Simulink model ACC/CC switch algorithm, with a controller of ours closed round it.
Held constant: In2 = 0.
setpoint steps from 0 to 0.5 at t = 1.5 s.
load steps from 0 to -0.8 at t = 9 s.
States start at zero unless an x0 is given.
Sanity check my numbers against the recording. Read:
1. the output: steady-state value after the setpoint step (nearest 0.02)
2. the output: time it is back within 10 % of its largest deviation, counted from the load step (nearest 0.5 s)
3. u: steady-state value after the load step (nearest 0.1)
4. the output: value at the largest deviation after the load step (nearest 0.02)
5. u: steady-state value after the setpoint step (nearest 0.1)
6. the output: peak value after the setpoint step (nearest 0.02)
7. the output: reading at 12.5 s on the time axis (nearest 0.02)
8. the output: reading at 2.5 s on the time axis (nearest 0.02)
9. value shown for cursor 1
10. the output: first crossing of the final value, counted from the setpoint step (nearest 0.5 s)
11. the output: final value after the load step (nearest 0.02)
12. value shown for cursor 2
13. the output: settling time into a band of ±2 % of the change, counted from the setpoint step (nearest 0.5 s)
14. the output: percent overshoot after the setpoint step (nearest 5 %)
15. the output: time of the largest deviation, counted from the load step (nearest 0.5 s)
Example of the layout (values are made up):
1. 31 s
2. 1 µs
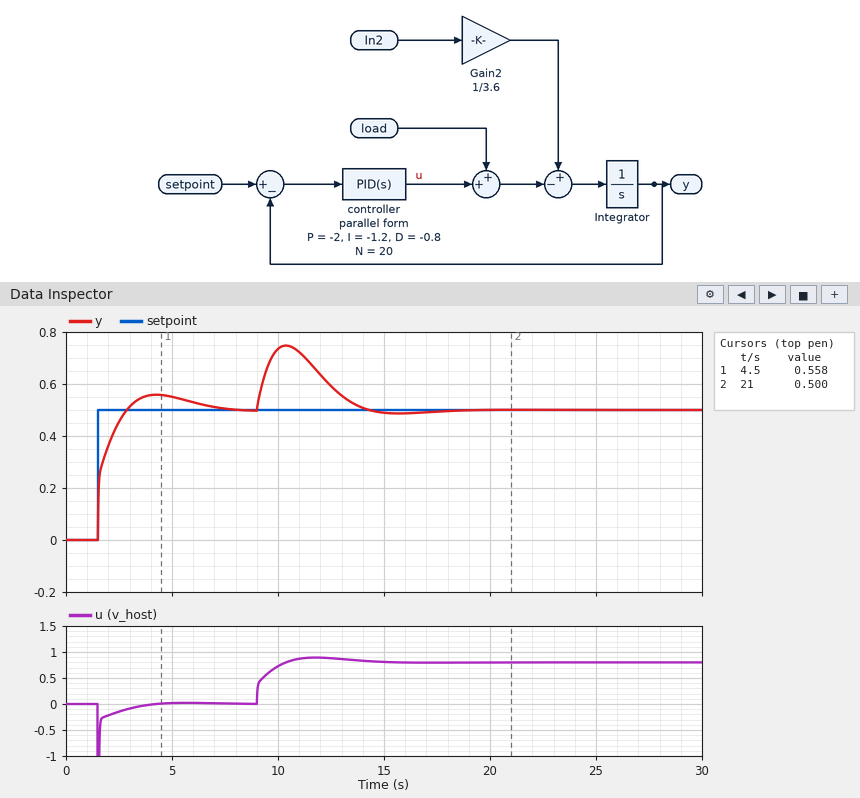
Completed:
1. 0.50
2. 4.5 s
3. 0.8
4. 0.74
5. 0.0
6. 0.56
7. 0.60
8. 0.46
9. 0.558
10. 1.5 s
11. 0.50
12. 0.500
13. 5.5 s
14. 10 %
15. 1.5 s
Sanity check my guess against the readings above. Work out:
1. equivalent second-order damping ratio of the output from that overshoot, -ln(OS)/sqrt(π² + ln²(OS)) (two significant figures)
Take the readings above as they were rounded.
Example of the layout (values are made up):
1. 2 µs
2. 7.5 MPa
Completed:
1. 0.59
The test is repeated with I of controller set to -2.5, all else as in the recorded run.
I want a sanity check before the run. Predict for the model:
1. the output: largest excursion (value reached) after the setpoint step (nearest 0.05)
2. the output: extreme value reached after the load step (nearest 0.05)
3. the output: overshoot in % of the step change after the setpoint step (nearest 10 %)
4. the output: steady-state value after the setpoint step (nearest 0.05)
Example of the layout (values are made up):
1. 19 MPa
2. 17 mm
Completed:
1. 0.60
2. 0.70
3. 20 %
4. 0.50
